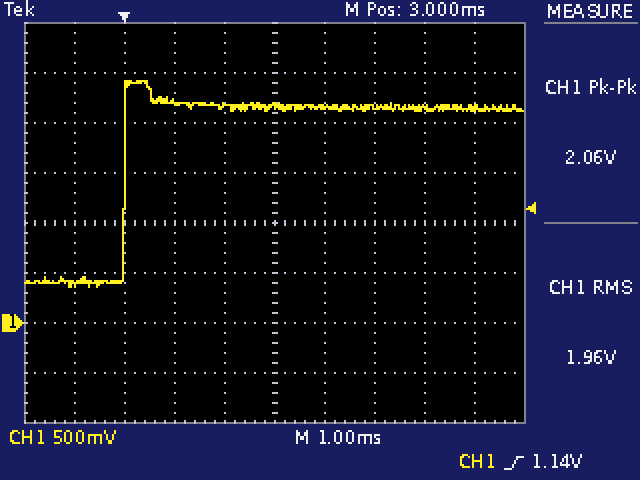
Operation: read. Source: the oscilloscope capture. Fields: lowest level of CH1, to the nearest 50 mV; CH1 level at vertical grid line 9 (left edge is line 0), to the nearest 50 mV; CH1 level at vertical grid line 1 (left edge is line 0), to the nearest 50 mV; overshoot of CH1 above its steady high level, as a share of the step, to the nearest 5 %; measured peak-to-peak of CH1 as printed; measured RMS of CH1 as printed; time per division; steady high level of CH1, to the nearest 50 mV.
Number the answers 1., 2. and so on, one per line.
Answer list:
1. 350 mV
2. 2.15 V
3. 400 mV
4. 15 %
5. 2.06 V
6. 1.96 V
7. 1 ms
8. 2.15 V
